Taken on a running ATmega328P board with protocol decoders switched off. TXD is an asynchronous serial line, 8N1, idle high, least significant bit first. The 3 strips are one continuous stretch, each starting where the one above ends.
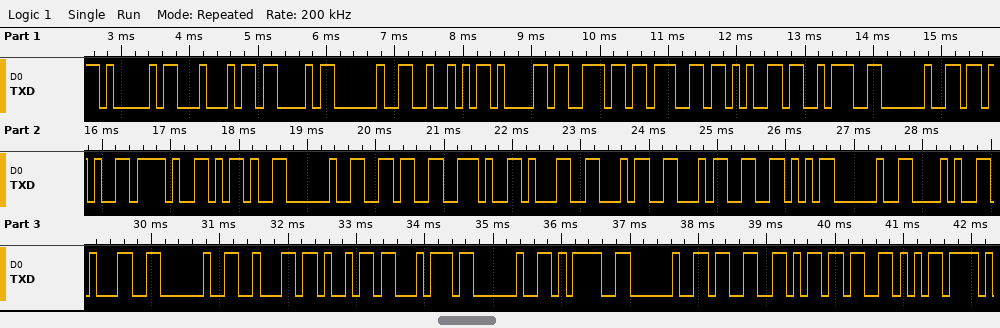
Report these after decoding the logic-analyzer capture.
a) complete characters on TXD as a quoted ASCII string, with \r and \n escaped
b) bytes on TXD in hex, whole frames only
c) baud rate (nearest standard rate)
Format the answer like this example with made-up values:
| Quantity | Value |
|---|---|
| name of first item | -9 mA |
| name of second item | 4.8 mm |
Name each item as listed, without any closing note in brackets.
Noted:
| Quantity | Value |
|---|---|
| complete characters on TXD as a quoted ASCII string, with \r and \n escaped | "ADC Range: +/- 6.144V (1 bit = 3mV" |
| bytes on TXD in hex, whole frames only | 41 44 43 20 52 61 6E 67 65 3A 20 2B 2F 2D 20 36 2E 31 34 34 56 20 28 31 20 62 69 74 20 3D 20 33 6D 56 |
| baud rate | 9600 baud |
